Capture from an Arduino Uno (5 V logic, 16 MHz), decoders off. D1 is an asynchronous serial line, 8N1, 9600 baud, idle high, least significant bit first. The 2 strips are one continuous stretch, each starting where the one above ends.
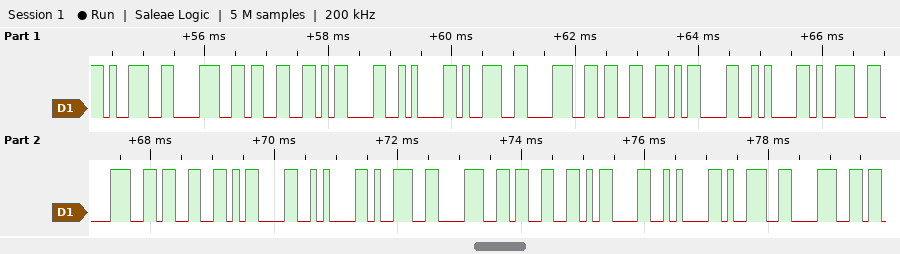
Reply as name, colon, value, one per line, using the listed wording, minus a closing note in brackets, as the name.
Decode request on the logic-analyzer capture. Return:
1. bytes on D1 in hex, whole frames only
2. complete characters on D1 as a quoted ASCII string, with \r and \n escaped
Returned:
bytes on D1 in hex, whole frames only: 39 38 33 0D 0A 39 38 33 0D 0A 39 38 33 0D 0A 39 38 33 0D 0A 39 38
complete characters on D1 as a quoted ASCII string, with \r and \n escaped: "983\r\n983\r\n983\r\n983\r\n98"
